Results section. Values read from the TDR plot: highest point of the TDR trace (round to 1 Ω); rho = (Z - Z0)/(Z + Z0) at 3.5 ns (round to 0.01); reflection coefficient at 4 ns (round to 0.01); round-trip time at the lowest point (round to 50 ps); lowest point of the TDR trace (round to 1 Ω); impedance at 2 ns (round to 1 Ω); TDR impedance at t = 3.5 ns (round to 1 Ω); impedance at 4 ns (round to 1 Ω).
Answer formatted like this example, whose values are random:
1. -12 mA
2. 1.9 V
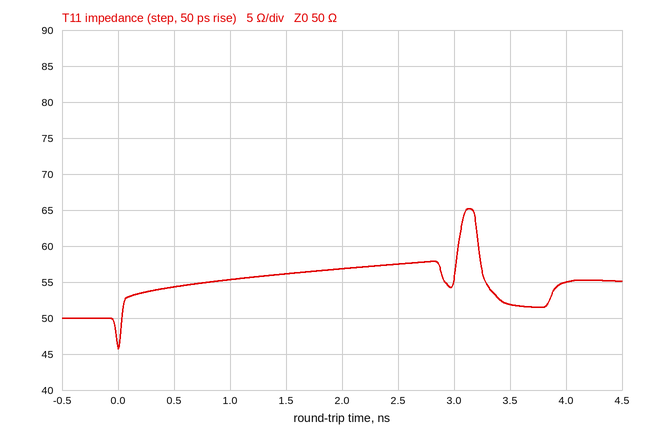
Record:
1. 65 Ω
2. +0.02
3. +0.05
4. 0 ps
5. 46 Ω
6. 57 Ω
7. 52 Ω
8. 55 Ω
